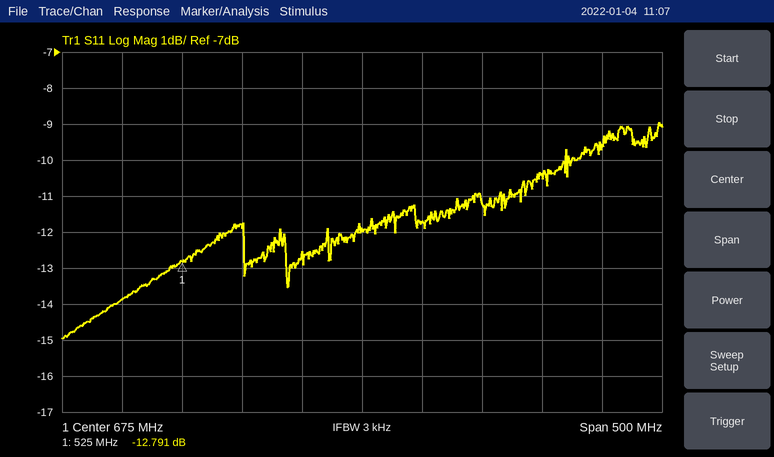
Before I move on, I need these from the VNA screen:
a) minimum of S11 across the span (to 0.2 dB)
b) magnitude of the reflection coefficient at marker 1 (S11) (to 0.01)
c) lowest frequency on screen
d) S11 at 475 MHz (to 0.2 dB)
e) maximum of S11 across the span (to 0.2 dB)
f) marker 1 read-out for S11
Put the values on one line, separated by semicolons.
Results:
-15.0 dB; 0.23; 425 MHz; -13.8 dB; -9.0 dB; -12.791 dB
